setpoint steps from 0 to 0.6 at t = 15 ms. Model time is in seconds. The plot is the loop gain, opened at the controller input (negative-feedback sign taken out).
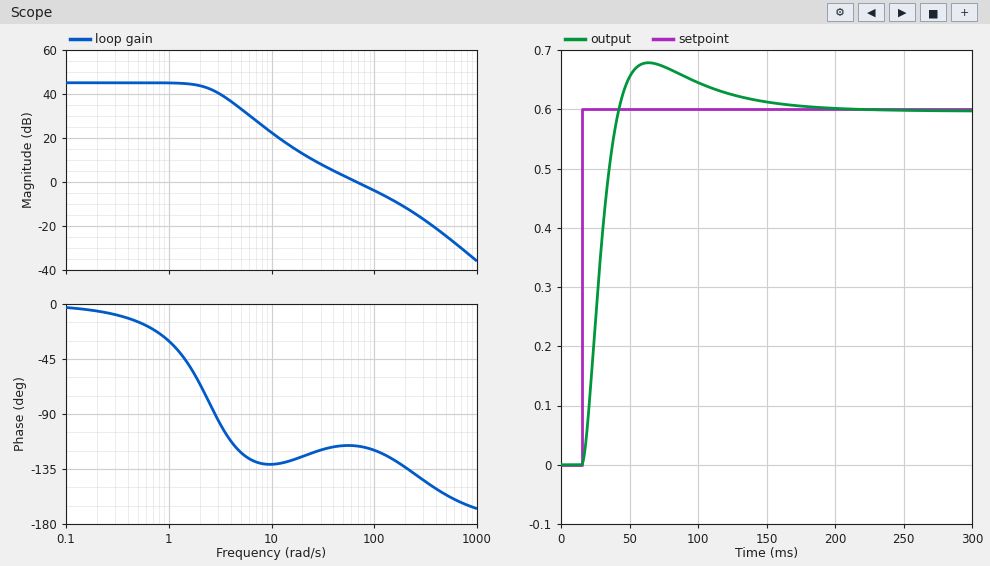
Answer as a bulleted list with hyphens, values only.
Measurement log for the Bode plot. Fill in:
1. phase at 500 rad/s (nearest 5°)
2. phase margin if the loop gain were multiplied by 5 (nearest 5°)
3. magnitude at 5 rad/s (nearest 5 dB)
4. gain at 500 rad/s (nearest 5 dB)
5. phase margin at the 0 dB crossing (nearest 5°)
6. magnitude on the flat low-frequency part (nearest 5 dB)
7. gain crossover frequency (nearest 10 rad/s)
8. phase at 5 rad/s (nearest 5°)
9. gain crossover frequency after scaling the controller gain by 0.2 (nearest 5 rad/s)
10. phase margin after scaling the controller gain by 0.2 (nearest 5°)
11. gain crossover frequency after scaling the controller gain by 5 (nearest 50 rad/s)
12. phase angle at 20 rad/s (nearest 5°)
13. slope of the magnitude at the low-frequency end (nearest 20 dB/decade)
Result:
- -155°
- 40°
- 35 dB
- -25 dB
- 65°
- 45 dB
- 70 rad/s
- -120°
- 20 rad/s
- 55°
- 250 rad/s
- -125°
- 0 dB/decade
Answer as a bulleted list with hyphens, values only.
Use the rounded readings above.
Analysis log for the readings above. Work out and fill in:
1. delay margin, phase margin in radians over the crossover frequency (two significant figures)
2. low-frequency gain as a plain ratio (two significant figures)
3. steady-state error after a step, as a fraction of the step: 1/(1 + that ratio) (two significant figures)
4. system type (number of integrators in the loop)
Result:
- 0.016 s
- 180
- 0.0055
- 0
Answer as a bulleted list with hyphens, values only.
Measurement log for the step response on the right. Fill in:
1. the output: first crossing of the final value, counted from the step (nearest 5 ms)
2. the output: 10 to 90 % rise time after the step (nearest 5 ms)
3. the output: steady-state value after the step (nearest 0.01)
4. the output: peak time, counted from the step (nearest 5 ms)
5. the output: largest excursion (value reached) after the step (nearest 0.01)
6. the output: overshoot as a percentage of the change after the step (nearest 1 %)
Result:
- 25 ms
- 20 ms
- 0.60
- 50 ms
- 0.68
- 14 %
